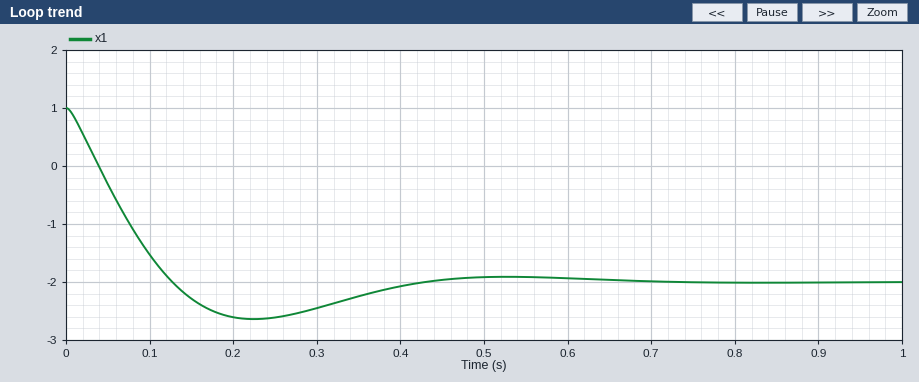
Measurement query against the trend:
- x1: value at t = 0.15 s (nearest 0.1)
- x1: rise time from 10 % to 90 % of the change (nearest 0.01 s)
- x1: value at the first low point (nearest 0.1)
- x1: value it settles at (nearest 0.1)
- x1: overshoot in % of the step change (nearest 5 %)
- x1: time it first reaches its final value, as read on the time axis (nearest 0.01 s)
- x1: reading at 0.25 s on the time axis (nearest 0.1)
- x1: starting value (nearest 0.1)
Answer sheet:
-2.3
0.09 s
-2.6
-2.0
20 %
0.13 s
-2.6
1.0
